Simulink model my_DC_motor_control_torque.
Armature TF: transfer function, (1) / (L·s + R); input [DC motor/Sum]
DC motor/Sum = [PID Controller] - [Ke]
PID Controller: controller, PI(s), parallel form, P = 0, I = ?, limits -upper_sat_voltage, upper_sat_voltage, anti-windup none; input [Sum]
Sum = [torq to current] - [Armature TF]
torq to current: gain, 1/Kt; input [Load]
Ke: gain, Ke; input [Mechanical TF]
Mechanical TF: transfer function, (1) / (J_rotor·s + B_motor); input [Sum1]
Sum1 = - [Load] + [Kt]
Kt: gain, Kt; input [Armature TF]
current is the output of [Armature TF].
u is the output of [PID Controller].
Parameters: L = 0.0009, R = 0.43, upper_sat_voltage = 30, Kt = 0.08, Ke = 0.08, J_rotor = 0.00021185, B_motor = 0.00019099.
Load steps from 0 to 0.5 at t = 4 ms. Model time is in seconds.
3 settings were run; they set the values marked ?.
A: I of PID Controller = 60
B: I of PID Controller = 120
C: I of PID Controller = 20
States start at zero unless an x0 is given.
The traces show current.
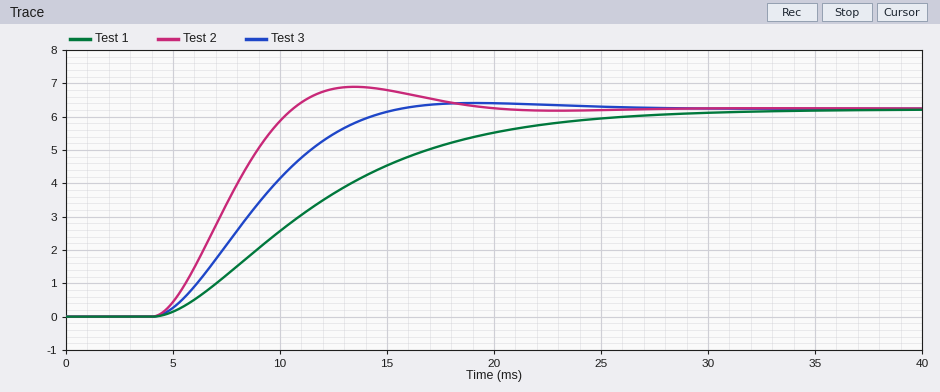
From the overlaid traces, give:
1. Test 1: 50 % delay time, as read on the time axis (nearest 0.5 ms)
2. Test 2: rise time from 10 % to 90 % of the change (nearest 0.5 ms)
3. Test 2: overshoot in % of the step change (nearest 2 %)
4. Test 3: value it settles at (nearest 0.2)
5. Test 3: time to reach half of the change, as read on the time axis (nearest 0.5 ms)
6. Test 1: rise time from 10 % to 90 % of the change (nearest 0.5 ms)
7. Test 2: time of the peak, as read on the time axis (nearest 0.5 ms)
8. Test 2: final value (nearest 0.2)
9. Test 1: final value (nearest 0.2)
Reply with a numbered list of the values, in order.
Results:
1. 11.0 ms
2. 4.5 ms
3. 10 %
4. 6.2
5. 8.5 ms
6. 14.5 ms
7. 13.5 ms
8. 6.2
9. 6.2
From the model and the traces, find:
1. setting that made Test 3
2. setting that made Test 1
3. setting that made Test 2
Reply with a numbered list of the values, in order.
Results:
1. A
2. C
3. B
